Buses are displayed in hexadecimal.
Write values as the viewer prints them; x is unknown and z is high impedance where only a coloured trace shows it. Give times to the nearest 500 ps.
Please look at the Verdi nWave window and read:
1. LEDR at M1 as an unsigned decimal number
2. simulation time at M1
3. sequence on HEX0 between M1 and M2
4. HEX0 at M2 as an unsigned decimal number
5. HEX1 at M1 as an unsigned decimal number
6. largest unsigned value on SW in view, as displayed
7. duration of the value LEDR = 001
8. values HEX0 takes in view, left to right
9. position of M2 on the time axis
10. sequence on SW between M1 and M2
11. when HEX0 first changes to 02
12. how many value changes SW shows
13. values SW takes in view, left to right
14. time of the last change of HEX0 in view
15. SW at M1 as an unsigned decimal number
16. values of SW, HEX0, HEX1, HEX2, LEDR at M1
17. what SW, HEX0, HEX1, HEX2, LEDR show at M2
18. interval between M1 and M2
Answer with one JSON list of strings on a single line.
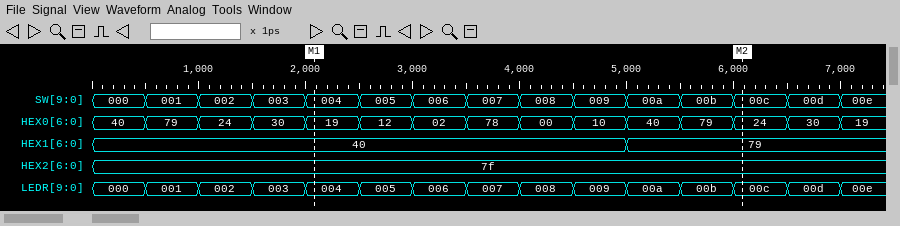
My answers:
["4", "2000 ps", "19, 12, 02, 78, 00, 10, 40, 79, 24", "36", "64", "00e", "500 ps", "40, 79, 24, 30, 19, 12, 02, 78, 00, 10, 40, 79, 24, 30, 19", "6000 ps", "004, 005, 006, 007, 008, 009, 00a, 00b, 00c", "3000 ps", "14", "000, 001, 002, 003, 004, 005, 006, 007, 008, 009, 00a, 00b, 00c, 00d, 00e", "7000 ps", "4", "SW=004, HEX0=19, HEX1=40, HEX2=7f, LEDR=004", "SW=00c, HEX0=24, HEX1=79, HEX2=7f, LEDR=00c", "4000 ps"]
